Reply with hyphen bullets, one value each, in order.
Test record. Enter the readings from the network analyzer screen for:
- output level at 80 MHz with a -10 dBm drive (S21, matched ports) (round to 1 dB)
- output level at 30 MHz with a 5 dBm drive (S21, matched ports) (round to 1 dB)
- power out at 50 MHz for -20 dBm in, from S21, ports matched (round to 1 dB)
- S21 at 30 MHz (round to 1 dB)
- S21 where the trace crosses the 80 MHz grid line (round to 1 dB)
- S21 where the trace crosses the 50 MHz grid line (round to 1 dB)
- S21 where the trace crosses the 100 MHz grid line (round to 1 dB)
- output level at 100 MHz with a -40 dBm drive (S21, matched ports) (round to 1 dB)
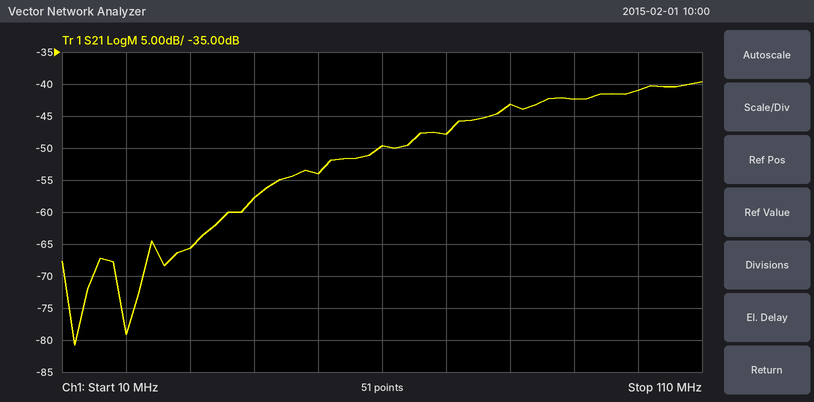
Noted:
- -53 dBm
- -61 dBm
- -74 dBm
- -66 dB
- -43 dB
- -54 dB
- -41 dB
- -81 dBm
